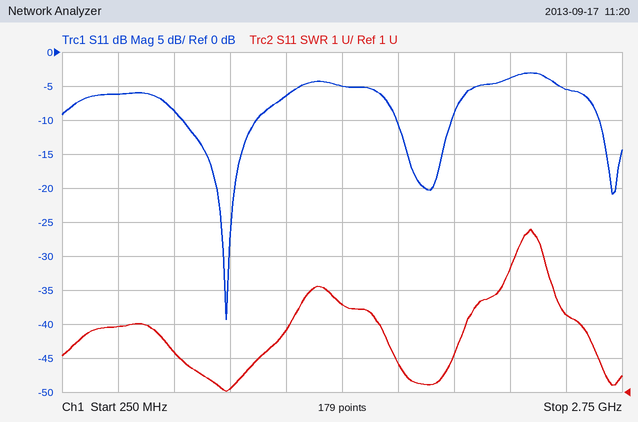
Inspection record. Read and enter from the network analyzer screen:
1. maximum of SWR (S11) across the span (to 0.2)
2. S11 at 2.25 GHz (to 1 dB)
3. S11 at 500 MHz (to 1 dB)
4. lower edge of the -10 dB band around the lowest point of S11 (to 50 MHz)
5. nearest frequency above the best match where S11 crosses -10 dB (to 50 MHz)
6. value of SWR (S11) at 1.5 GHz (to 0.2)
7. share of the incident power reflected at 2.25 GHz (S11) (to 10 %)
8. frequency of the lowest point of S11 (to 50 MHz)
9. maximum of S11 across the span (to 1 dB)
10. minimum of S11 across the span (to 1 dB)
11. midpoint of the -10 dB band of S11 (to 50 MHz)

5.8
-4 dB
-6 dB
800 MHz
1.10 GHz
3.6
40 %
1.00 GHz
-3 dB
-39 dB
950 MHz
